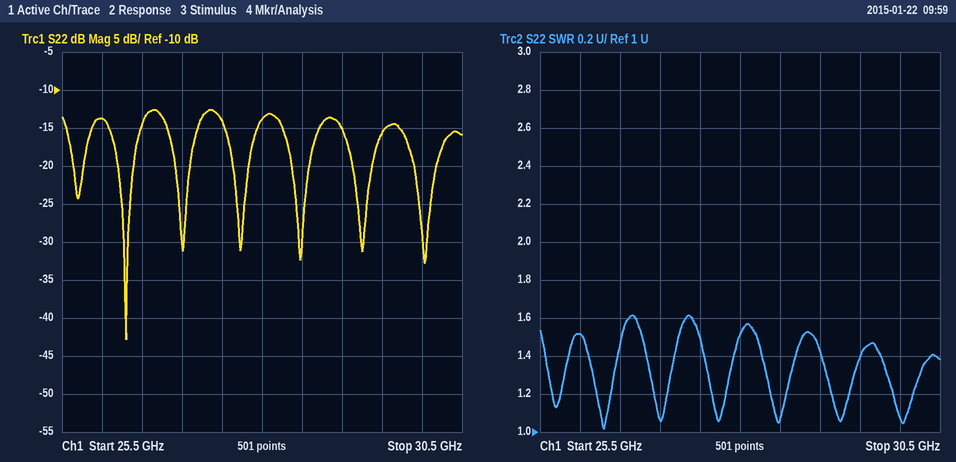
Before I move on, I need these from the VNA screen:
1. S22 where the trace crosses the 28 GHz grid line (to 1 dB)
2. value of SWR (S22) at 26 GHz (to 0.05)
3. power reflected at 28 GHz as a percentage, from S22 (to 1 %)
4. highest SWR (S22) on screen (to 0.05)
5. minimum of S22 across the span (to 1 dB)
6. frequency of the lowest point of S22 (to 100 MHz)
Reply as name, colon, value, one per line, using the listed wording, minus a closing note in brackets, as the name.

S22 where the trace crosses the 28 GHz grid line: -14 dB
value of SWR (S22) at 26 GHz: 1.50
power reflected at 28 GHz as a percentage, from S22: 4 %
highest SWR (S22) on screen: 1.60
minimum of S22 across the span: -43 dB
frequency of the lowest point of S22: 26.3 GHz
